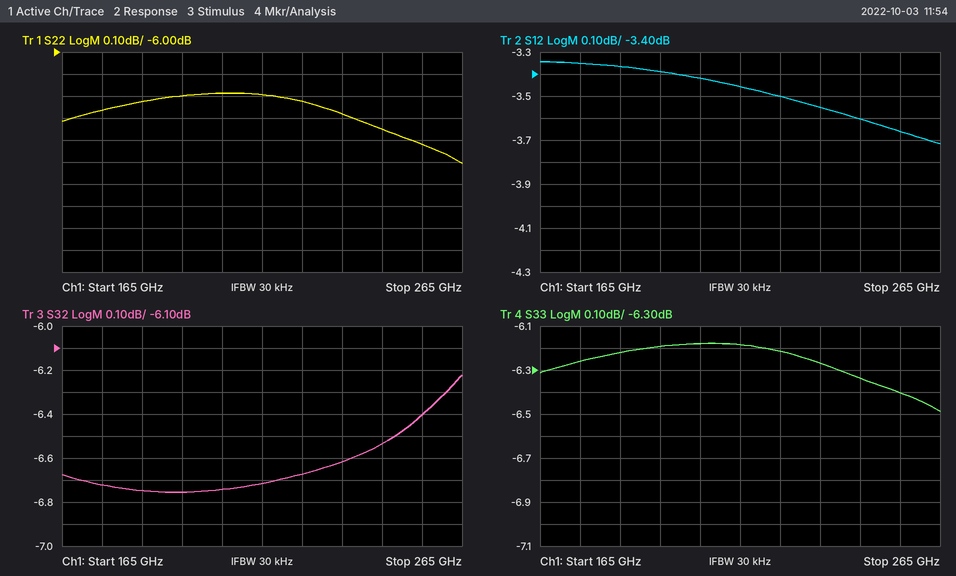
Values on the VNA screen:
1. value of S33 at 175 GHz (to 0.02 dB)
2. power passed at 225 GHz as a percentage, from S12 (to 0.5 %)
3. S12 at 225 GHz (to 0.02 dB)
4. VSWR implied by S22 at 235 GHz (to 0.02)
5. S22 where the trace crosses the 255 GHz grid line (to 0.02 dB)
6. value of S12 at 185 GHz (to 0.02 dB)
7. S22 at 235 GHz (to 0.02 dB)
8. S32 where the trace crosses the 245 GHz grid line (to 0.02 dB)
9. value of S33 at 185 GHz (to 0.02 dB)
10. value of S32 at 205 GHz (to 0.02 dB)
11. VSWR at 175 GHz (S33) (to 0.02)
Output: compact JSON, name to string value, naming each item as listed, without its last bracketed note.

{"value of S33 at 175 GHz": "-6.26 dB", "power passed at 225 GHz as a percentage, from S12": "44.5 %", "S12 at 225 GHz": "-3.50 dB", "VSWR implied by S22 at 235 GHz": "2.88", "S22 where the trace crosses the 255 GHz grid line": "-6.42 dB", "value of S12 at 185 GHz": "-3.36 dB", "S22 at 235 GHz": "-6.28 dB", "S32 where the trace crosses the 245 GHz grid line": "-6.54 dB", "value of S33 at 185 GHz": "-6.22 dB", "value of S32 at 205 GHz": "-6.74 dB", "VSWR at 175 GHz (S33)": "2.90"}
